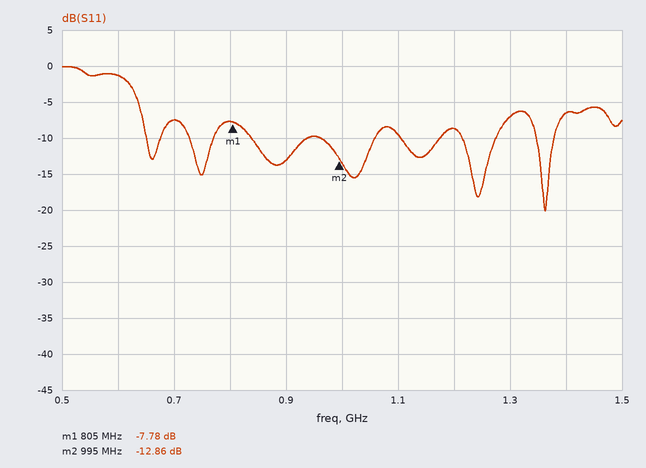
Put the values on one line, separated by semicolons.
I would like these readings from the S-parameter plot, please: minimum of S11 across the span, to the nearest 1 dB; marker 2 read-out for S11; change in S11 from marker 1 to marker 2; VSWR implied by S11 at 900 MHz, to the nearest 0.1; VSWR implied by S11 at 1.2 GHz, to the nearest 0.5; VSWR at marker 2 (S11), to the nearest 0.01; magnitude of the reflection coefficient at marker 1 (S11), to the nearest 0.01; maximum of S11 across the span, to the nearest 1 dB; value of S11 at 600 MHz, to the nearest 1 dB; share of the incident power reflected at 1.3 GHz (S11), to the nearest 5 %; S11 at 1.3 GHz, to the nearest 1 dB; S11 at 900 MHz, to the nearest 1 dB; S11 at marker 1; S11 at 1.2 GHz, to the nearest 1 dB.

-20 dB; -12.86 dB; -5.08 dB; 1.6; 2.0; 1.59; 0.41; 0 dB; -1 dB; 20 %; -7 dB; -13 dB; -7.78 dB; -9 dB
